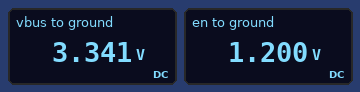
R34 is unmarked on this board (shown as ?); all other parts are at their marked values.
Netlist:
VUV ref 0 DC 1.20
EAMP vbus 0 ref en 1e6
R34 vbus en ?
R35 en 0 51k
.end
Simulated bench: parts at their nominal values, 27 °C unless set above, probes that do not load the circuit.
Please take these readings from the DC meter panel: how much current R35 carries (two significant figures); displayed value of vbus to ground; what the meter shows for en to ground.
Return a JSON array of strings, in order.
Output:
["24 µA", "3.341 V", "1.200 V"]
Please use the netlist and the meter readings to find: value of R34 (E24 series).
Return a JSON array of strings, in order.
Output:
["91 kΩ"]
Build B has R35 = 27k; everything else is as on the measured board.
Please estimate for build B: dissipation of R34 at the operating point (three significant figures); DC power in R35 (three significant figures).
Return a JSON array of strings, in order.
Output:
["180 µW", "53.3 µW"]
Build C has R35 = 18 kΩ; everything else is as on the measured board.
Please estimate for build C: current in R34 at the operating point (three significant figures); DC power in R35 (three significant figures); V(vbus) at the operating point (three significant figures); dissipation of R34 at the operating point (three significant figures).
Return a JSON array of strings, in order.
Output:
["66.7 µA", "80.0 µW", "7.27 V", "404 µW"]
